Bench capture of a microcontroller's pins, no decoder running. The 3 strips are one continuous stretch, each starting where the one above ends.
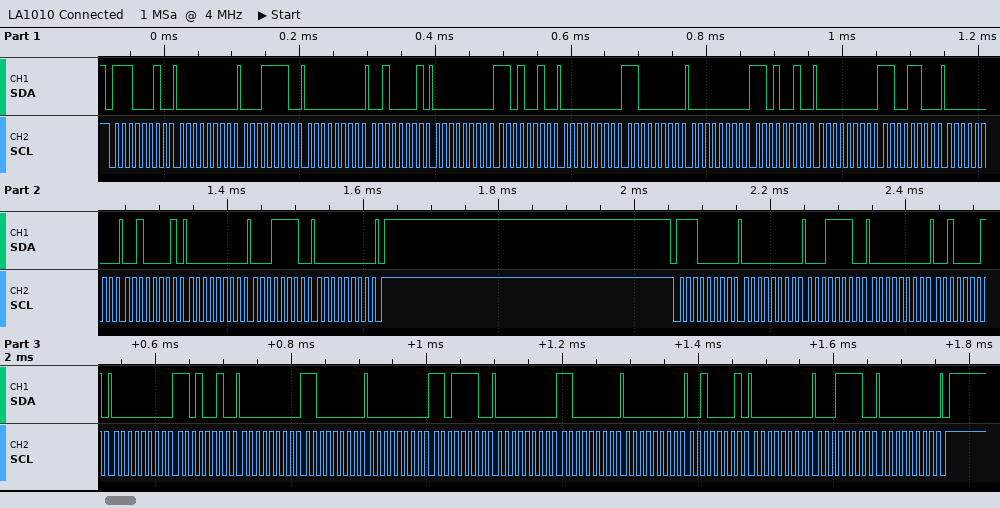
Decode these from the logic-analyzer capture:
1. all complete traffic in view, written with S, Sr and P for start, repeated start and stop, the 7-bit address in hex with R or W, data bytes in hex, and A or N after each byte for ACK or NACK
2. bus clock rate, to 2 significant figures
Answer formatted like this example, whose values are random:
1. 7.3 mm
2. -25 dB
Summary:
1. S 71W A 00 A 1E A 00 A 21 A 00 A D2 A 00 A C0 A 00 A D2 A 00 A CC A 00 A 21 A 00 A 1E A 00 A P S 70W A 00 A 1E A 00 A 21 A 00 A D2 A 00 A C0 A 00 A DE A 00 A C0 A 00 A 21 A 00 A 1E A 00 A P
2. 100 kHz
